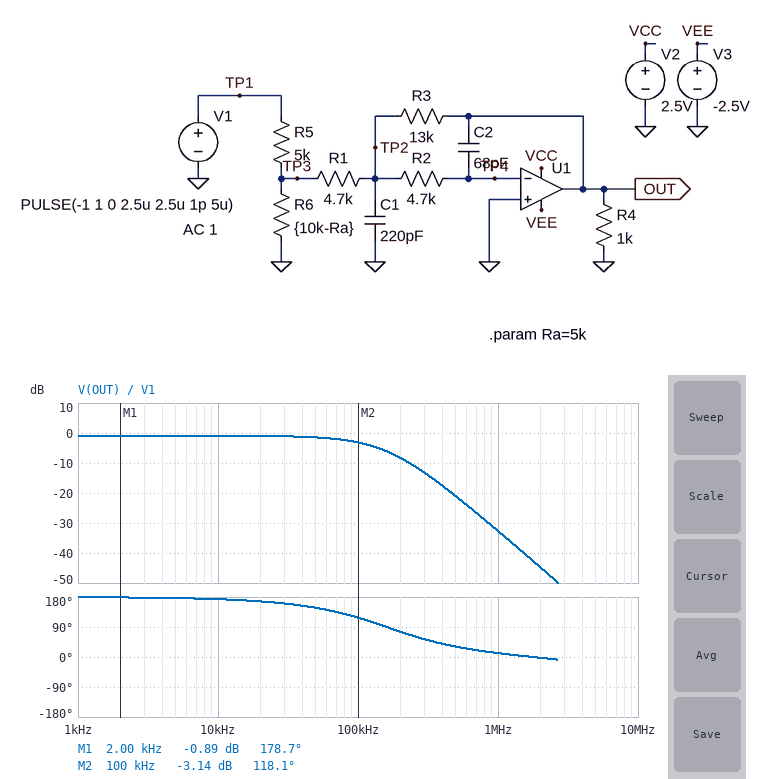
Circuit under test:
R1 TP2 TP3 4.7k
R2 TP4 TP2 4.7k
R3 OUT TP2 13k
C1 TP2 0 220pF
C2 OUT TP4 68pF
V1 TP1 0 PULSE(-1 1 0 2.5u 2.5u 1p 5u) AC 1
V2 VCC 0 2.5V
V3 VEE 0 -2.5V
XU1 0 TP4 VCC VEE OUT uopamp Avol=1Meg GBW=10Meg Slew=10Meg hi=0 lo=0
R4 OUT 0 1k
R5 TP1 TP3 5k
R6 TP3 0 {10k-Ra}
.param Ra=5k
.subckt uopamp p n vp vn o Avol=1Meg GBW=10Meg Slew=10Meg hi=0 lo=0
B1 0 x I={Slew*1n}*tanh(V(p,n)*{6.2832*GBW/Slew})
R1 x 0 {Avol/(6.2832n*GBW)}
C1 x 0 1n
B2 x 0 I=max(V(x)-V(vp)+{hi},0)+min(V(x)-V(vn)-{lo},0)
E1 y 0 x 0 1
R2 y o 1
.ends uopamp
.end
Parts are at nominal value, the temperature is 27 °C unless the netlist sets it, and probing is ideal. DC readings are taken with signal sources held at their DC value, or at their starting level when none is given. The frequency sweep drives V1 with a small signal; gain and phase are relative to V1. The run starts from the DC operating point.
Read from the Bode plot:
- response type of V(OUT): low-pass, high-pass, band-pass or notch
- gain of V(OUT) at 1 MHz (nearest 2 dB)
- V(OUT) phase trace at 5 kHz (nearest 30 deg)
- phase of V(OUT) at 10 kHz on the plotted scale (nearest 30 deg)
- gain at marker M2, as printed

low-pass
-32 dB
180 deg
180 deg
-3.14 dB
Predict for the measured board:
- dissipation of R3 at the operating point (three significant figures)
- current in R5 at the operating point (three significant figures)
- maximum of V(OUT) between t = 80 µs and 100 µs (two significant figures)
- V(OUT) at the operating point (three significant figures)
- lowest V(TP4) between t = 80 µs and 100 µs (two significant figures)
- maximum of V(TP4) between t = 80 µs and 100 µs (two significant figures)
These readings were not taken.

62.7 µW
135 µA
310 mV
903 mV
-6.7 mV
6.7 mV
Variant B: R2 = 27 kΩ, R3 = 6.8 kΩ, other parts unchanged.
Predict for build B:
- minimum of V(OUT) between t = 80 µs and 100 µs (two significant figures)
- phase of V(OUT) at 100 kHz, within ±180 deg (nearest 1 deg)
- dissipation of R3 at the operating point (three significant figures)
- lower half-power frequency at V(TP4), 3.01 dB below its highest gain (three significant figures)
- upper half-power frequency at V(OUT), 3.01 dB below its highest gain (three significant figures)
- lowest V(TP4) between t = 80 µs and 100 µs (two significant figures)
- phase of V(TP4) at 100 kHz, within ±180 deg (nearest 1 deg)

-62 mV
87 deg
32.8 µW
34.3 kHz
46.9 kHz
-1.3 mV
-3 deg
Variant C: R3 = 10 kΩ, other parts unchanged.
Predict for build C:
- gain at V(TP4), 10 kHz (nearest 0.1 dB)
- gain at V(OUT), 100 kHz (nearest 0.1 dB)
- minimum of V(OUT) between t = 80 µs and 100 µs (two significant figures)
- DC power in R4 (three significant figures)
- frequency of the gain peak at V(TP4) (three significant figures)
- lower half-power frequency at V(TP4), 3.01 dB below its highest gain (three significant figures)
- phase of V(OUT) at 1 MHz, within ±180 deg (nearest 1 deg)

-63.2 dB
-4.5 dB
-300 mV
482 µW
185 kHz
85.4 kHz
13 deg
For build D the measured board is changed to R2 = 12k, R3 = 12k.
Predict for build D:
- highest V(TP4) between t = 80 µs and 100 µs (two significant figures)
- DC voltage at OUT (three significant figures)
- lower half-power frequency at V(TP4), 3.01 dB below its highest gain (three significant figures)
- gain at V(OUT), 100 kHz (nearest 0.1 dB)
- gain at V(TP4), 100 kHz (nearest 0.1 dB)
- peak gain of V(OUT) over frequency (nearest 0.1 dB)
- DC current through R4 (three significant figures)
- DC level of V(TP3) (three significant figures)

3.1 mV
833 mV
43.9 kHz
-7.2 dB
-47.2 dB
-1.6 dB
833 µA
-326 mV
